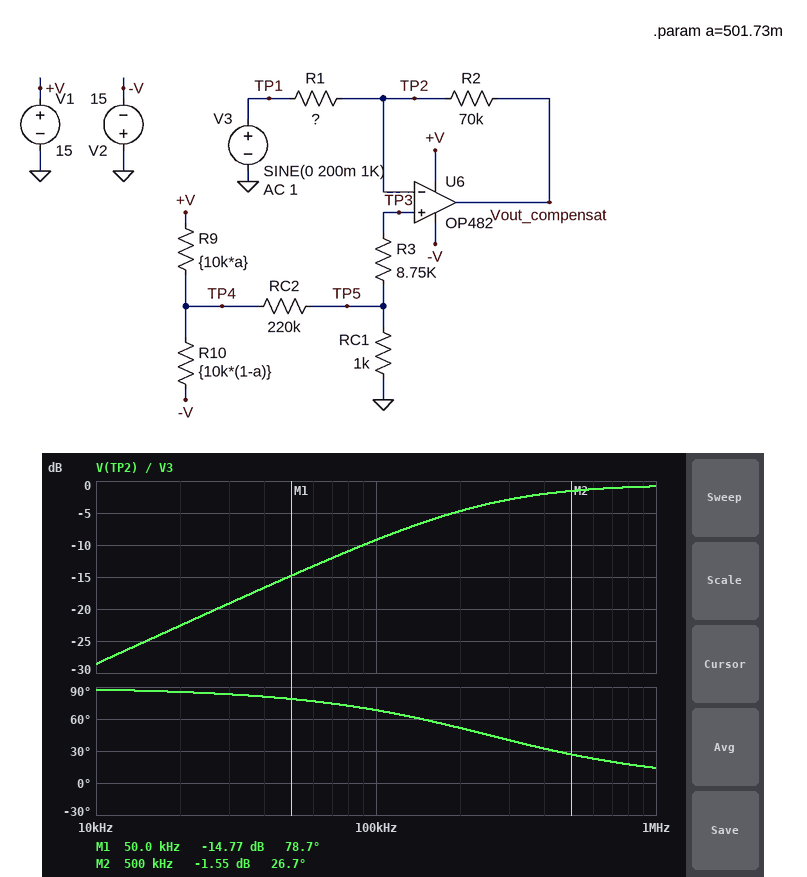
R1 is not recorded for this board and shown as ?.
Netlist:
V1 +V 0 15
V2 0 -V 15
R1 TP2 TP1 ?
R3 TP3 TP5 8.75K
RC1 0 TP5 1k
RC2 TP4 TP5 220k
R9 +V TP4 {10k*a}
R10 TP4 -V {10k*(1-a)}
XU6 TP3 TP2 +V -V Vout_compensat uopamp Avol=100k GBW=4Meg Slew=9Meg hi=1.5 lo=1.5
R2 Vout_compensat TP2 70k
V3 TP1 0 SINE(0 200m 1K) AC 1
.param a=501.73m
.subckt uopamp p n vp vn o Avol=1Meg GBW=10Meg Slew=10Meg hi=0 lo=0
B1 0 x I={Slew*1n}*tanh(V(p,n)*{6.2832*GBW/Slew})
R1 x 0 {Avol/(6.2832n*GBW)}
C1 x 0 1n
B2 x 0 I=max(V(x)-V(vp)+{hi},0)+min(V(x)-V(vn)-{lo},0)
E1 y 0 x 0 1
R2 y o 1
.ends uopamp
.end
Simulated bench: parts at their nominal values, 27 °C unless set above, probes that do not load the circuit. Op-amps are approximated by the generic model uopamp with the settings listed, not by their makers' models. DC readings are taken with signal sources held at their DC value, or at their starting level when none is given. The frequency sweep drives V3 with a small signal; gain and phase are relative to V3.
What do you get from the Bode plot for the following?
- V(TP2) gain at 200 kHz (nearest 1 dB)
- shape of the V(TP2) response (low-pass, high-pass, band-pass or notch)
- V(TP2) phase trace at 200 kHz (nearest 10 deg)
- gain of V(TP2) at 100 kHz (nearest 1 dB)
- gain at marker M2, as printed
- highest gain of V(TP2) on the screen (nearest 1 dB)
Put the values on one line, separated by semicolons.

-5 dB; high-pass; 50 deg; -9 dB; -1.55 dB; -1 dB
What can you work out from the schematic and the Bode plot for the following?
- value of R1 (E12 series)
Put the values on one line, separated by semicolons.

4.7 kΩ
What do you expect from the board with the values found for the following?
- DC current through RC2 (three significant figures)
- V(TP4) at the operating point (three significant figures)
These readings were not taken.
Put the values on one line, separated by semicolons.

232 nA; -51.3 mV
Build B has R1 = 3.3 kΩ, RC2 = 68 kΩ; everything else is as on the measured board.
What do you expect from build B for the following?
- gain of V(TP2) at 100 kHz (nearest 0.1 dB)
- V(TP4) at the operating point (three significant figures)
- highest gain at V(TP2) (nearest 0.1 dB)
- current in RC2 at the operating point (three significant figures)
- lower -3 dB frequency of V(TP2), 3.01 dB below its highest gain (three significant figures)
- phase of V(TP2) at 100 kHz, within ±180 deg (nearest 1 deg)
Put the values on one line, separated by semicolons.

-6.7 dB; -50.1 mV; -0.4 dB; 726 nA; 180 kHz; 61 deg
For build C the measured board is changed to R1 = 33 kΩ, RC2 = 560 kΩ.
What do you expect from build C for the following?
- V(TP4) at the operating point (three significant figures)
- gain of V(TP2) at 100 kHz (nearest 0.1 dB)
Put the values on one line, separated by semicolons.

-51.7 mV; -25.5 dB
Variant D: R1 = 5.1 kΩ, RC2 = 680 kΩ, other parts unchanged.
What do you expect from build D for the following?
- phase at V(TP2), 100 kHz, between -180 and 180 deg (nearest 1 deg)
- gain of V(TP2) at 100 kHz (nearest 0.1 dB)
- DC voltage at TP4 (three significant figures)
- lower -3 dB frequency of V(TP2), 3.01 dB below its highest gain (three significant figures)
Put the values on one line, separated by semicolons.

70 deg; -9.8 dB; -51.7 mV; 272 kHz
